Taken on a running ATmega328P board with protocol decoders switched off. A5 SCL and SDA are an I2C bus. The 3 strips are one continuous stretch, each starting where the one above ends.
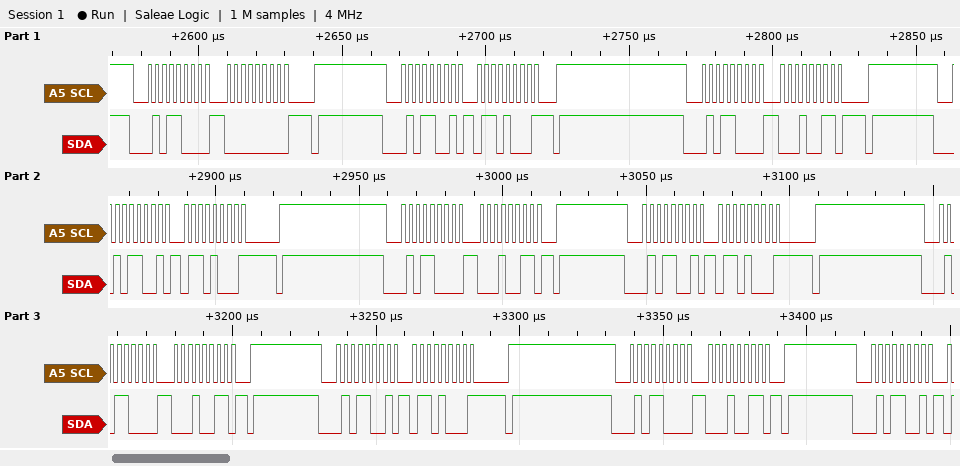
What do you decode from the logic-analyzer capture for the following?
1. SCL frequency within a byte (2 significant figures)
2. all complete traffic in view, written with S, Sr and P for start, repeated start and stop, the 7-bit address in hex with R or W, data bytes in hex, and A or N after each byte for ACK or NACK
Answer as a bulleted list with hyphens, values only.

- 400 kHz
- S 2CW A 00 A P S 2CR A 68 N P S 2CW A 13 A P S 2CR A 68 N P S 2CW A 13 A P S 2CR A 68 N P S 2CW A 13 A P S 2CR A 68 N P S 2CW A 13 A P S 2CR A
